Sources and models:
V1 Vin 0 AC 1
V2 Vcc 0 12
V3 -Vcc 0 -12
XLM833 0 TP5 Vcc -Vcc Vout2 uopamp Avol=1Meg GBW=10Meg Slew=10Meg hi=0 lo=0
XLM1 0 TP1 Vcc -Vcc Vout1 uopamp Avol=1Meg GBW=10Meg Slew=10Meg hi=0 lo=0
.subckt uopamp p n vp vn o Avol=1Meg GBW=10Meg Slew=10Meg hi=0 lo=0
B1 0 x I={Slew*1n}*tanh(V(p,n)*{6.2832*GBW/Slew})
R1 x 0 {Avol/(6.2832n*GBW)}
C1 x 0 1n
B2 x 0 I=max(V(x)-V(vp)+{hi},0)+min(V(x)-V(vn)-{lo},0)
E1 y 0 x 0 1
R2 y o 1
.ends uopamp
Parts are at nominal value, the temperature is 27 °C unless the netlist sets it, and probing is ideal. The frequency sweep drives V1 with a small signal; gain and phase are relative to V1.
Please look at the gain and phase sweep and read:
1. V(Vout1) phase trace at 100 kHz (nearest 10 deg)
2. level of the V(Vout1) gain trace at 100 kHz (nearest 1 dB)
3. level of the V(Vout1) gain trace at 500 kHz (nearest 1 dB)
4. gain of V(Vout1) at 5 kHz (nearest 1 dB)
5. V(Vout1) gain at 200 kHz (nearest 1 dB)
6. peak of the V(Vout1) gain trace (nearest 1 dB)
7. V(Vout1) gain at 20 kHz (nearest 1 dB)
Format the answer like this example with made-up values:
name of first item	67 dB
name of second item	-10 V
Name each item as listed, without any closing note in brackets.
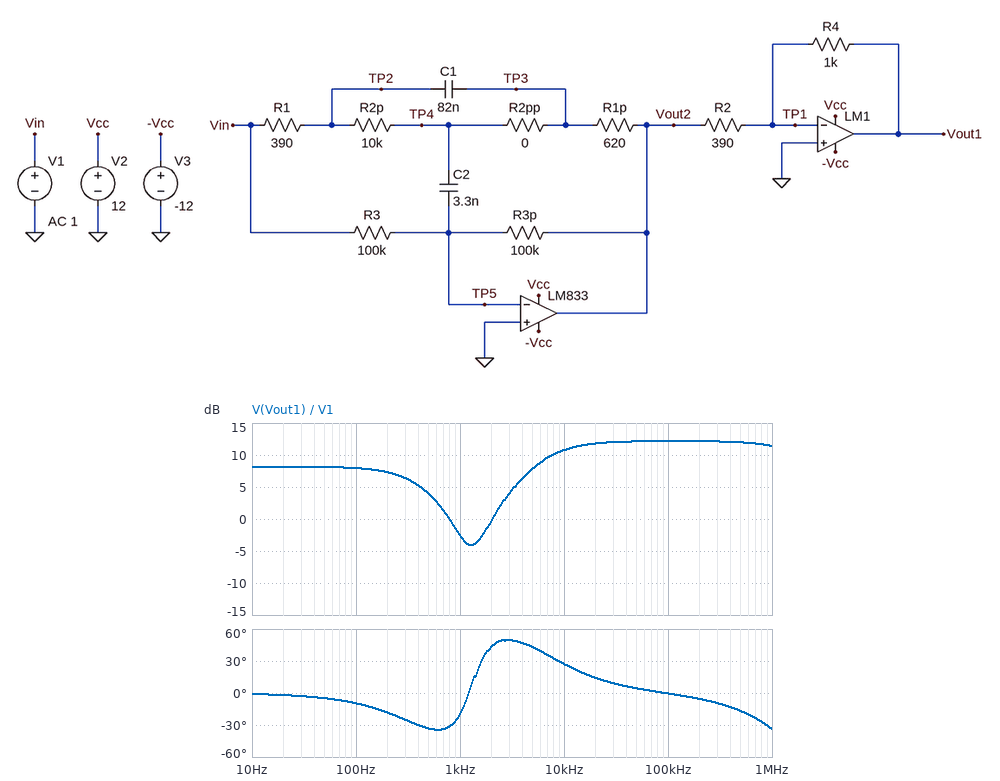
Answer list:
V(Vout1) phase trace at 100 kHz	0 deg
level of the V(Vout1) gain trace at 100 kHz	12 dB
level of the V(Vout1) gain trace at 500 kHz	12 dB
gain of V(Vout1) at 5 kHz	8 dB
V(Vout1) gain at 200 kHz	12 dB
peak of the V(Vout1) gain trace	12 dB
V(Vout1) gain at 20 kHz	12 dB
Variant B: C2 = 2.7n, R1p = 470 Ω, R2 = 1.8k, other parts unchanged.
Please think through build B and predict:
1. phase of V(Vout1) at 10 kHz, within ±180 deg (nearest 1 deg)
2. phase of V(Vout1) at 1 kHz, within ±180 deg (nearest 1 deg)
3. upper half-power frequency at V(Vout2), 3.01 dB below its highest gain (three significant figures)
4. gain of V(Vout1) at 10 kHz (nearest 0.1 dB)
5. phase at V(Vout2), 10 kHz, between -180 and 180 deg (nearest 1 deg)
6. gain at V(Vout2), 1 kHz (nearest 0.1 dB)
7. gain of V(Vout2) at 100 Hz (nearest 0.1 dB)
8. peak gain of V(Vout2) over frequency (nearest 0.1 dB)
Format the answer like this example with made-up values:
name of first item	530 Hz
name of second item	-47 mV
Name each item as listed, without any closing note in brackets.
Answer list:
phase of V(Vout1) at 10 kHz, within ±180 deg	26 deg
phase of V(Vout1) at 1 kHz, within ±180 deg	-33 deg
upper half-power frequency at V(Vout2), 3.01 dB below its highest gain	4.71 MHz
gain of V(Vout1) at 10 kHz	-4.9 dB
phase at V(Vout2), 10 kHz, between -180 and 180 deg	-154 deg
gain at V(Vout2), 1 kHz	-8.7 dB
gain of V(Vout2) at 100 Hz	-0.2 dB
peak gain of V(Vout2) over frequency	1.6 dB
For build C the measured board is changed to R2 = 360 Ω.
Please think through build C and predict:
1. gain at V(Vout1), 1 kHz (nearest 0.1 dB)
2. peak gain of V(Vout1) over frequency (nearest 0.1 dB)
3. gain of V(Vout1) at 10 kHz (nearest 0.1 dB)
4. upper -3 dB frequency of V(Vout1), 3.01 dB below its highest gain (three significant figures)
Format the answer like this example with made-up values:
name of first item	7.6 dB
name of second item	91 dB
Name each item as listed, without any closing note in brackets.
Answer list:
gain at V(Vout1), 1 kHz	-1.9 dB
peak gain of V(Vout1) over frequency	12.9 dB
gain of V(Vout1) at 10 kHz	11.5 dB
upper -3 dB frequency of V(Vout1), 3.01 dB below its highest gain	2.02 MHz
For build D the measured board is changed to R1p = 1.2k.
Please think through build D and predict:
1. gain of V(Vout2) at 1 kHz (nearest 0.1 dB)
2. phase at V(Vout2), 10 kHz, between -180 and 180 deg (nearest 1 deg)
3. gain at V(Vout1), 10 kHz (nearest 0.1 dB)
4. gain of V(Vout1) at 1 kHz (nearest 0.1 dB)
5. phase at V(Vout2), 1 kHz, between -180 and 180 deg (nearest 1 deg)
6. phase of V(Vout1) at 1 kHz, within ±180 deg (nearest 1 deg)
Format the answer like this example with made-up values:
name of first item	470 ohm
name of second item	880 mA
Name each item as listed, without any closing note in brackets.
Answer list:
gain of V(Vout2) at 1 kHz	-9.0 dB
phase at V(Vout2), 10 kHz, between -180 and 180 deg	-149 deg
gain at V(Vout1), 10 kHz	16.2 dB
gain of V(Vout1) at 1 kHz	-0.8 dB
phase at V(Vout2), 1 kHz, between -180 and 180 deg	-163 deg
phase of V(Vout1) at 1 kHz, within ±180 deg	17 deg
